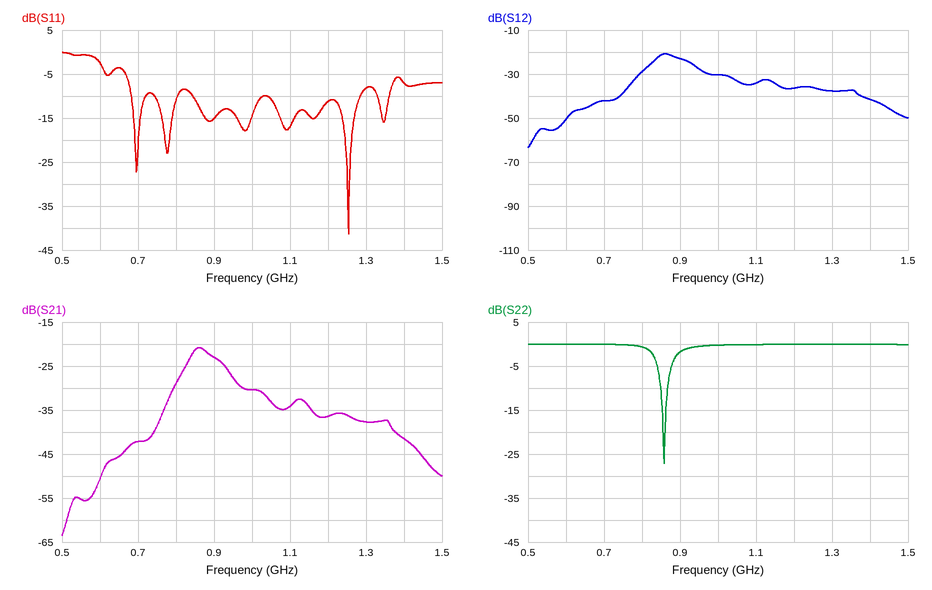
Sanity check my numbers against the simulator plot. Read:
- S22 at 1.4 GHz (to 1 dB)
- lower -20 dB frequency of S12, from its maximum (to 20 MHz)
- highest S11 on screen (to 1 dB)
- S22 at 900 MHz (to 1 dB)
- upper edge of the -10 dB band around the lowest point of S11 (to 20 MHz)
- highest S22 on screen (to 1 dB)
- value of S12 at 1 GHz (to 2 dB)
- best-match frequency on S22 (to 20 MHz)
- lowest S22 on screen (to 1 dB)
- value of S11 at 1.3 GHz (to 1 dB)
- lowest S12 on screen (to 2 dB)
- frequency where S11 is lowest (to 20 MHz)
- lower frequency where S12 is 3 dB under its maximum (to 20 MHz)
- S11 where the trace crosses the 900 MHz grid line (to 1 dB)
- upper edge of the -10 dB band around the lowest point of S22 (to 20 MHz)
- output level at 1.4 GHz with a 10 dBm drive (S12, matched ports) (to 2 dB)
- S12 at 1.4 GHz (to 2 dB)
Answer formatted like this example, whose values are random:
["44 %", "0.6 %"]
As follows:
["0 dB", "740 MHz", "0 dB", "-2 dB", "1.28 GHz", "0 dB", "-30 dB", "860 MHz", "-27 dB", "-8 dB", "-64 dB", "1.26 GHz", "840 MHz", "-15 dB", "860 MHz", "-32 dBm", "-42 dB"]
